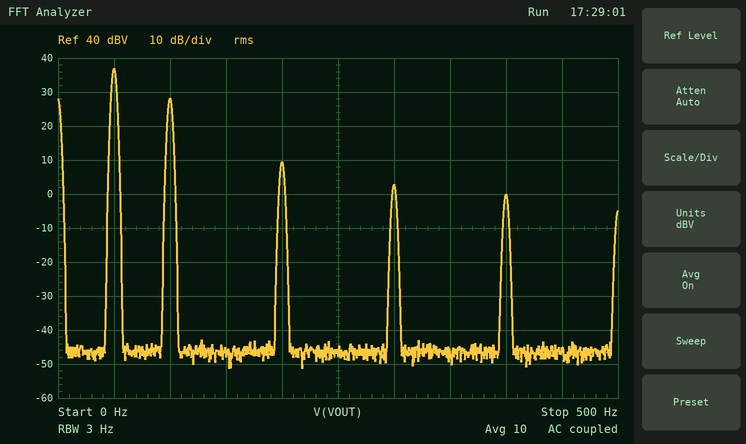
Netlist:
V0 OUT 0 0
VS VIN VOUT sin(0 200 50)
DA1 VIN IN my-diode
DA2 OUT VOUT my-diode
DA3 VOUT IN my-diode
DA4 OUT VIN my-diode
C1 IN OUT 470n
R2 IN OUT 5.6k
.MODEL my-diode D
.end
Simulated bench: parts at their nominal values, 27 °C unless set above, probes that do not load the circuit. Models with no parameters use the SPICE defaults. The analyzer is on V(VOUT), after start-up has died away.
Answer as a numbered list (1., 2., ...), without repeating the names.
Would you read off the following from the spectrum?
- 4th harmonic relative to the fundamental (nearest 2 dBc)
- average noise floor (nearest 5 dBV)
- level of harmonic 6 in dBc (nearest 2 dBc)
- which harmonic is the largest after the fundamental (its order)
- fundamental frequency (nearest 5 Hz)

1. -28 dBc
2. -45 dBV
3. -34 dBc
4. 2
5. 50 Hz
